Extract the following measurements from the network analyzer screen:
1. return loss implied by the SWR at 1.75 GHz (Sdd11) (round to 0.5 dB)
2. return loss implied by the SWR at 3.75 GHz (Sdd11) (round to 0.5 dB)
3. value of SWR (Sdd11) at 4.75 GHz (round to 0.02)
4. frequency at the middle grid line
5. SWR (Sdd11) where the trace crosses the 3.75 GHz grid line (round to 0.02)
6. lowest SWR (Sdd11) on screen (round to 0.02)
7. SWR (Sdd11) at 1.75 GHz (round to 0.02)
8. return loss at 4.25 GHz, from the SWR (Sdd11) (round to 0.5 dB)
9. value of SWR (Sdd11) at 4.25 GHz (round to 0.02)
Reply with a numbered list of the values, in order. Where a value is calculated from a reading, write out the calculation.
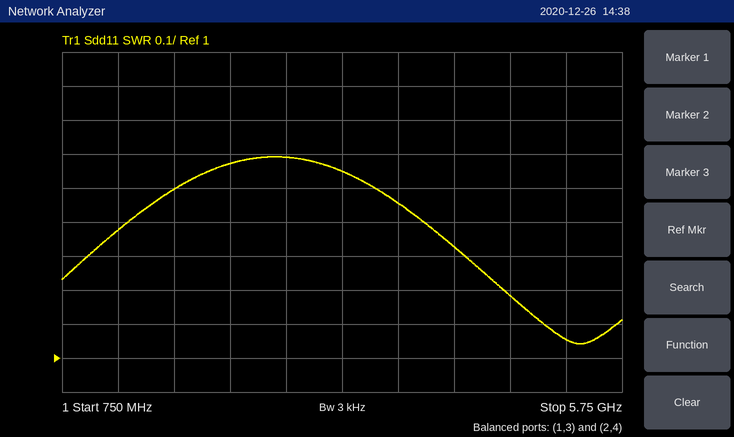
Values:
1. −20 log10((1.5 − 1)/(1.5 + 1)) ≈ 14.0 dB
2. −20 log10((1.46 − 1)/(1.46 + 1)) ≈ 14.6 dB, so 14.5 dB to the nearest 0.5 dB
3. 1.18
4. 3.25 GHz
5. 1.46
6. 1.04
7. 1.50
8. −20 log10((1.32 − 1)/(1.32 + 1)) ≈ 17.2 dB, so 17.0 dB to the nearest 0.5 dB
9. 1.32
